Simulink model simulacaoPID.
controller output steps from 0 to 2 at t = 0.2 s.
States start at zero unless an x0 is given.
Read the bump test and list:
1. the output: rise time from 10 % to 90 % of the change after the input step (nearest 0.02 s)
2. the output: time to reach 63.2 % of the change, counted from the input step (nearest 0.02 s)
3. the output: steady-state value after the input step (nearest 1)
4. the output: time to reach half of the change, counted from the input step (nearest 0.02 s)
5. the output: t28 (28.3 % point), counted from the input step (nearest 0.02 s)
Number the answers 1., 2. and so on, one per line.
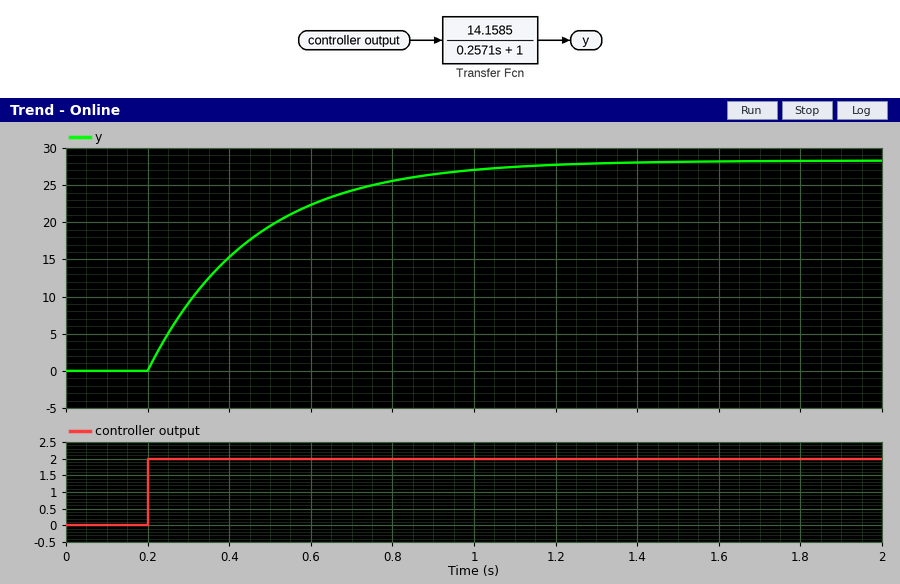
1. 0.56 s
2. 0.26 s
3. 28
4. 0.18 s
5. 0.08 s
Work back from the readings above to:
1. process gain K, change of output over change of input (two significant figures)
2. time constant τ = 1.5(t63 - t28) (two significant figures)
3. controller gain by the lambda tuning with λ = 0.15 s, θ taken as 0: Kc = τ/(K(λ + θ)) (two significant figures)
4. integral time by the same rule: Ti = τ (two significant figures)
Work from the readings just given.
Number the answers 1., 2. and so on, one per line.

1. 14
2. 0.27 s
3. 0.13
4. 0.27 s
